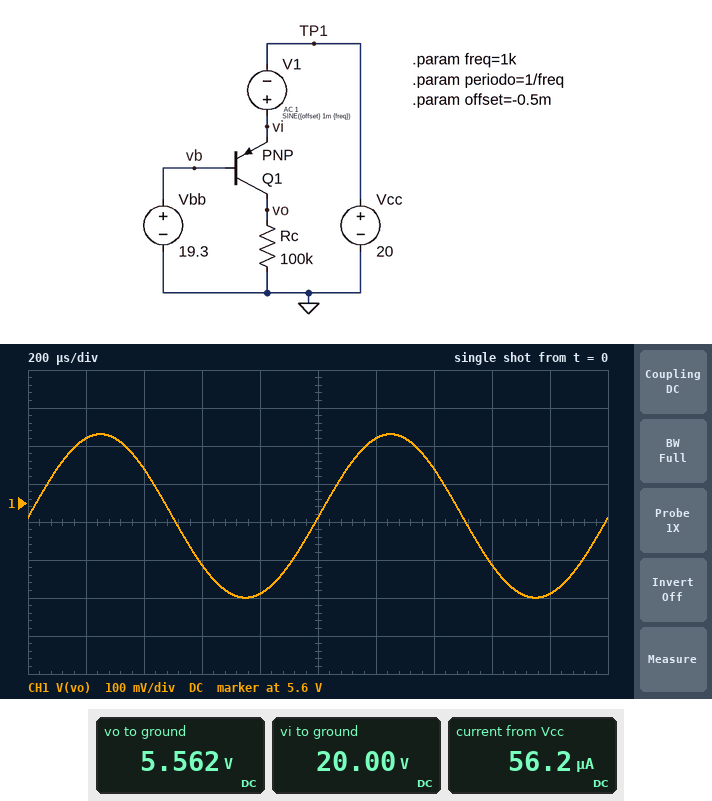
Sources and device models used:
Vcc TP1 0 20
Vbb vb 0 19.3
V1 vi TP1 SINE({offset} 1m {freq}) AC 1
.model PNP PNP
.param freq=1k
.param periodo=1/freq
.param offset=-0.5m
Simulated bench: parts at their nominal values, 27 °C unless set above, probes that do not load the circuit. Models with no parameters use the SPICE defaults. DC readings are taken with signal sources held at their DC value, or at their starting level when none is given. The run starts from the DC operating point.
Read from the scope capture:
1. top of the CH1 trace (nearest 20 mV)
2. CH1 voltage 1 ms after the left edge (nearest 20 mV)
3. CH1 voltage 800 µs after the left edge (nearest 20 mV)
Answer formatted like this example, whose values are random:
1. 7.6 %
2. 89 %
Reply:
1. 5.78 V
2. 5.56 V
3. 5.36 V
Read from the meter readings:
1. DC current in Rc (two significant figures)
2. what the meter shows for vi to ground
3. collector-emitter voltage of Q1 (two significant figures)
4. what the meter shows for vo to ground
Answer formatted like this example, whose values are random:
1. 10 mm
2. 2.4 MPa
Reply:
1. 56 µA
2. 20.00 V
3. -14 V
4. 5.562 V
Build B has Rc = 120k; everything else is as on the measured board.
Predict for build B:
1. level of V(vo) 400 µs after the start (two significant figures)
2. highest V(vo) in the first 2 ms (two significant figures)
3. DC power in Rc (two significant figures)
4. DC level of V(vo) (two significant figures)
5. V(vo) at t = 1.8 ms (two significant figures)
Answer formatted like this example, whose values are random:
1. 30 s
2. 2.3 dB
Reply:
1. 6.8 V
2. 6.9 V
3. 370 µW
4. 6.7 V
5. 6.4 V
